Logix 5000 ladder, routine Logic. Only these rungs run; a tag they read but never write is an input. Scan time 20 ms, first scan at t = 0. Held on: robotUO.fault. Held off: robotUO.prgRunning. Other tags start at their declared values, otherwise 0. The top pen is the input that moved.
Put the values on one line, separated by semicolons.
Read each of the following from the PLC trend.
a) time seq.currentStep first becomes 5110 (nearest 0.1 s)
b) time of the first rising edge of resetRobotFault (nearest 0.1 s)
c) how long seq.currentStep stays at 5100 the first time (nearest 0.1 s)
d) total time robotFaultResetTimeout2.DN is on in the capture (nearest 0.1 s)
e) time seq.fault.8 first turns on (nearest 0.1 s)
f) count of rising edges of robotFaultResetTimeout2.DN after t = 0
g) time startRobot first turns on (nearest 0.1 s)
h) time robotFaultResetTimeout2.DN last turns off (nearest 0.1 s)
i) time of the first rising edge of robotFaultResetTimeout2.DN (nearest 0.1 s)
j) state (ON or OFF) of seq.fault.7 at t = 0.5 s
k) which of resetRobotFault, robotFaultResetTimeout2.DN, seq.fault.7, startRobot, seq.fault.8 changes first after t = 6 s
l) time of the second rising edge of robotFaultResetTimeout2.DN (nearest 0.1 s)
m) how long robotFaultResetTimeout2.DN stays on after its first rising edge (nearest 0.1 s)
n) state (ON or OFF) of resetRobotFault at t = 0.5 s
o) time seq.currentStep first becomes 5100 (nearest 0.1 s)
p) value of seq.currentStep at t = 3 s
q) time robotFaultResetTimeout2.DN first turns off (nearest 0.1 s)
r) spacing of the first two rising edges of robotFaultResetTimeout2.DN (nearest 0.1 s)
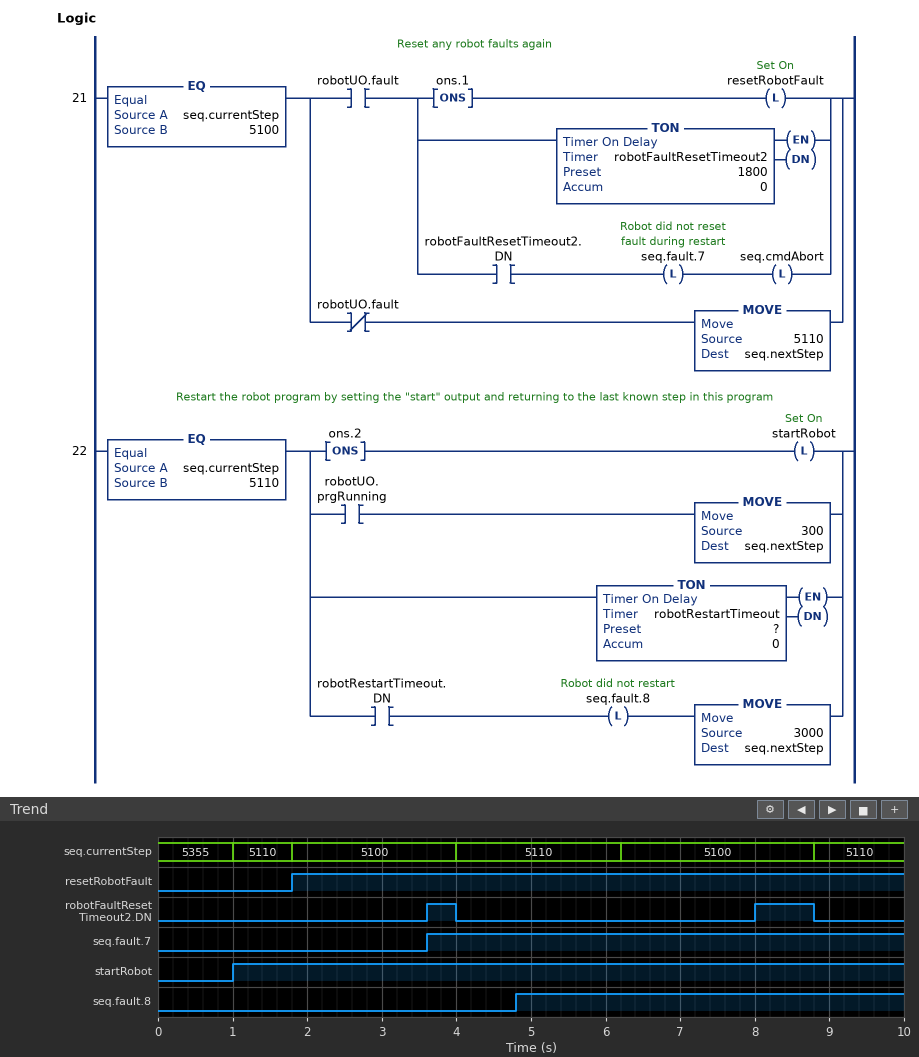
1.0 s; 1.8 s; 2.2 s; 1.2 s; 4.8 s; 2; 1.0 s; 8.8 s; 3.6 s; OFF; robotFaultResetTimeout2.DN; 8.0 s; 0.4 s; OFF; 1.8 s; 5100; 4.0 s; 4.4 s
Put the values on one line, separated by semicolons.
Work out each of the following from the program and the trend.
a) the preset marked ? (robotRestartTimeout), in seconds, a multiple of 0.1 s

0.8 s
